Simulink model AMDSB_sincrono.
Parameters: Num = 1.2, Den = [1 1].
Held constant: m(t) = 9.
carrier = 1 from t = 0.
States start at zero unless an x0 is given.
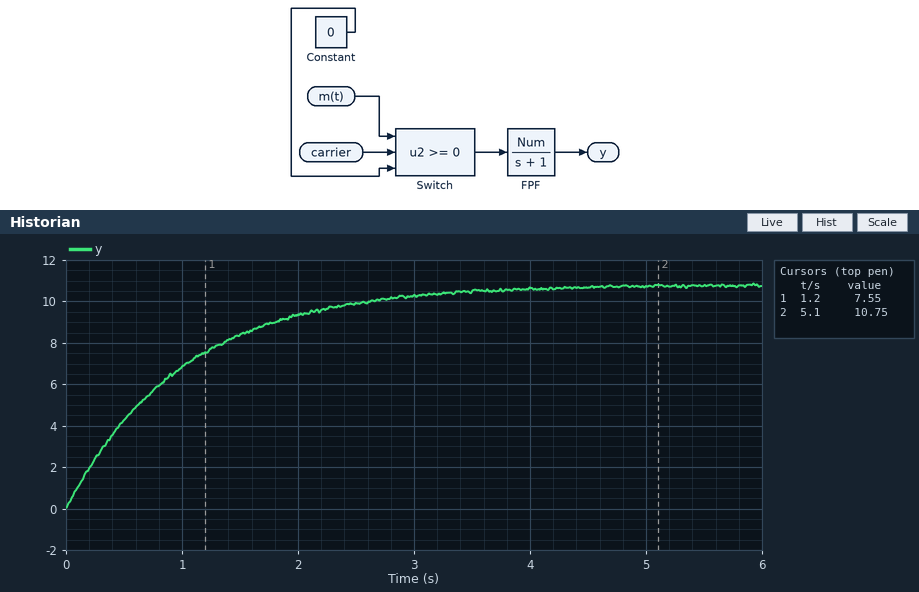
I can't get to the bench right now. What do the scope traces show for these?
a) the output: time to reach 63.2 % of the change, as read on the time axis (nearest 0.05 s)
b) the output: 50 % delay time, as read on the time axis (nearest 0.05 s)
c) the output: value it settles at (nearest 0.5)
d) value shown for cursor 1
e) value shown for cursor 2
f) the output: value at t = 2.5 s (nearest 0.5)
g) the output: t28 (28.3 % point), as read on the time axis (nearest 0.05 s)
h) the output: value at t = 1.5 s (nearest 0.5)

1.00 s
0.70 s
11.0
7.55
10.75
10.0
0.35 s
8.5
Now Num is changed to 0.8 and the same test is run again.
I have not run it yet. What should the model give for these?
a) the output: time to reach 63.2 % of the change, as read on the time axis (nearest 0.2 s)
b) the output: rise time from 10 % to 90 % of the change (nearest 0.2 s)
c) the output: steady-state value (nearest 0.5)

1.0 s
2.2 s
7.0
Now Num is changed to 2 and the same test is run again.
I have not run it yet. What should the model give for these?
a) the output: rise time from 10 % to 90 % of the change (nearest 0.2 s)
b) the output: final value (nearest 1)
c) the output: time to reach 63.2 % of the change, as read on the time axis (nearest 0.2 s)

2.2 s
18
1.0 s
